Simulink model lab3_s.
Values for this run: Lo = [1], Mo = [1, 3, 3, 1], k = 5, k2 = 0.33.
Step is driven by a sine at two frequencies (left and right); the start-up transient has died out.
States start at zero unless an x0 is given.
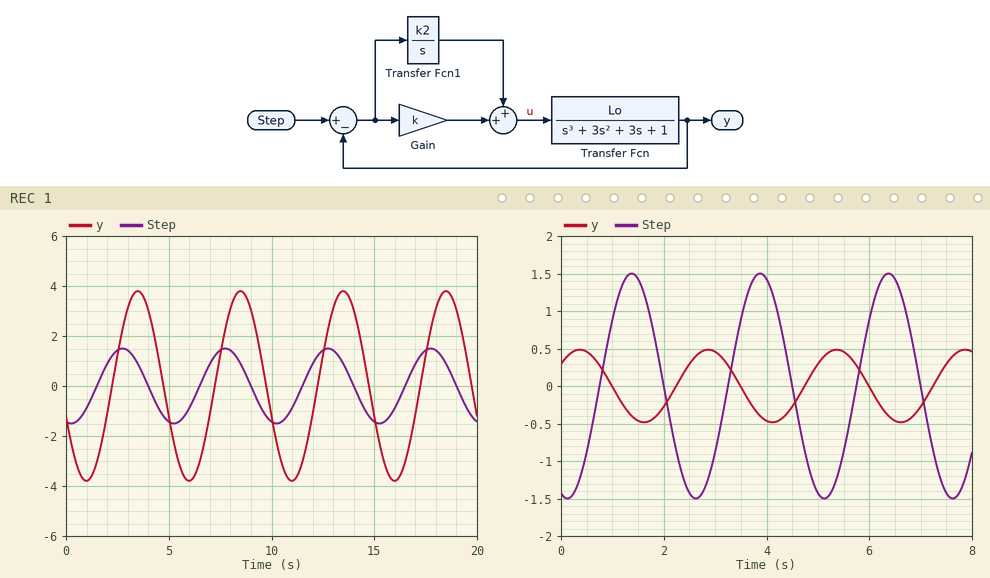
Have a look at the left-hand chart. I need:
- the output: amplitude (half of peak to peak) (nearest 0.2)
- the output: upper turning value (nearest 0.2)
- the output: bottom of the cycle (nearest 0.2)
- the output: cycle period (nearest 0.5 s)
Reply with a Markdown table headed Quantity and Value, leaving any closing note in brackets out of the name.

| Quantity | Value |
|---|---|
| the output: amplitude (half of peak to peak) | 3.8 |
| the output: upper turning value | 3.8 |
| the output: bottom of the cycle | -3.8 |
| the output: cycle period | 5.0 s |
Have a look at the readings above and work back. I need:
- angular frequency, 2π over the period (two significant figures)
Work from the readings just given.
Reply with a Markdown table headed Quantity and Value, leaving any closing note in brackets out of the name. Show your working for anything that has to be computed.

| Quantity | Value |
|---|---|
| angular frequency, 2π over the period | 2π / 5 = 1.3 rad/s |
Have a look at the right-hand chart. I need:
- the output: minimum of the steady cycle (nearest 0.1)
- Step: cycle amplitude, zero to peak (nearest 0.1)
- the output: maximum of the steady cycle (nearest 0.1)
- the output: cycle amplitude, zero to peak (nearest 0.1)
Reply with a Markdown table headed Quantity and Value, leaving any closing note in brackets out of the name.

| Quantity | Value |
|---|---|
| the output: minimum of the steady cycle | -0.5 |
| Step: cycle amplitude, zero to peak | 1.5 |
| the output: maximum of the steady cycle | 0.5 |
| the output: cycle amplitude, zero to peak | 0.5 |
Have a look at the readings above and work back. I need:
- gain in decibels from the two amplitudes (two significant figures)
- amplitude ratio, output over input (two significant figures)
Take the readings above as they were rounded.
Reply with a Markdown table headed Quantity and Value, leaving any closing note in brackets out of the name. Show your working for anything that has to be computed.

| Quantity | Value |
|---|---|
| gain in decibels from the two amplitudes | 20 log10(0.5 / 1.5) = -9.5 dB |
| amplitude ratio, output over input | 0.5 / 1.5 = 0.33 |
